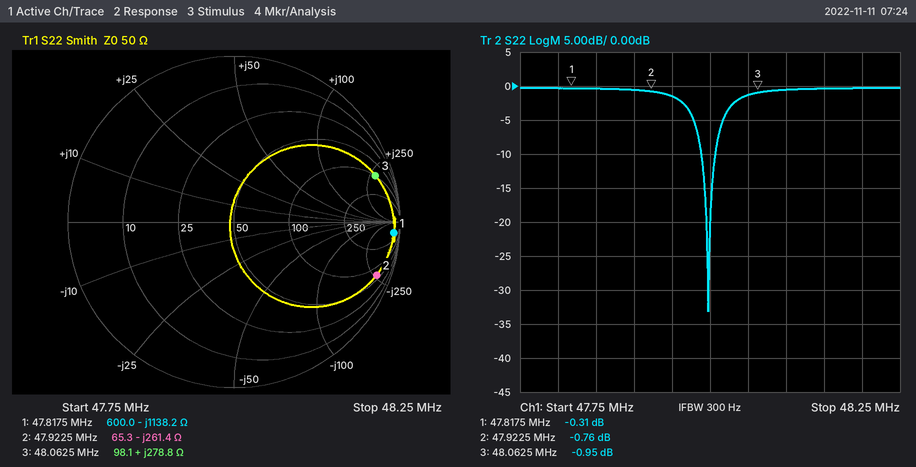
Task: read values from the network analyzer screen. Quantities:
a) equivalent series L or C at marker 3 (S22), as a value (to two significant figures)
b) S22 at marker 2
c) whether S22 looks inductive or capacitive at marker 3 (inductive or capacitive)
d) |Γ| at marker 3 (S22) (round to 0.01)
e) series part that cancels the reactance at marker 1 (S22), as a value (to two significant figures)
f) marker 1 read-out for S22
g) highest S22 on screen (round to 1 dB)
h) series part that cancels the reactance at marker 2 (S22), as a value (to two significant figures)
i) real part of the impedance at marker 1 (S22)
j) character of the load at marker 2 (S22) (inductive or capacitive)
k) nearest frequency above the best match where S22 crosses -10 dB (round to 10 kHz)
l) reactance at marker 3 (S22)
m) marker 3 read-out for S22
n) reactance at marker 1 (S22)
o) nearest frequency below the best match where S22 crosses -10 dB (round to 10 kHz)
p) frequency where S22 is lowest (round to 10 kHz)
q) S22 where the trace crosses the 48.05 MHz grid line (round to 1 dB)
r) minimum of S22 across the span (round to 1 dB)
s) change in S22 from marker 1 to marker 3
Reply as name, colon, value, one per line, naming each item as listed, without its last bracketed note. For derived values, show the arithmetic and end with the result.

equivalent series L or C at marker 3 (S22), as a value: L = 278.8 Ω/(2π × 48.0625 MHz) ≈ 923 nH, so 920 nH to two significant figures
S22 at marker 2: -0.76 dB
whether S22 looks inductive or capacitive at marker 3: inductive
|Γ| at marker 3 (S22): 0.90
series part that cancels the reactance at marker 1 (S22), as a value: L = 1138.2 Ω/(2π × 47.8175 MHz) ≈ 3.8 µH
marker 1 read-out for S22: -0.31 dB
highest S22 on screen: 0 dB
series part that cancels the reactance at marker 2 (S22), as a value: L = 261.4 Ω/(2π × 47.9225 MHz) ≈ 868 nH, so 870 nH to two significant figures
real part of the impedance at marker 1: 600.0 Ω
character of the load at marker 2 (S22): capacitive
nearest frequency above the best match where S22 crosses -10 dB: 48.01 MHz
reactance at marker 3: +278.8 Ω
marker 3 read-out for S22: -0.95 dB
reactance at marker 1: -1138.2 Ω
nearest frequency below the best match where S22 crosses -10 dB: 47.99 MHz
frequency where S22 is lowest: 48.00 MHz
S22 where the trace crosses the 48.05 MHz grid line: -1 dB
minimum of S22 across the span: -33 dB
change in S22 from marker 1 to marker 3: -0.95 − (-0.31) = -0.64 dB
